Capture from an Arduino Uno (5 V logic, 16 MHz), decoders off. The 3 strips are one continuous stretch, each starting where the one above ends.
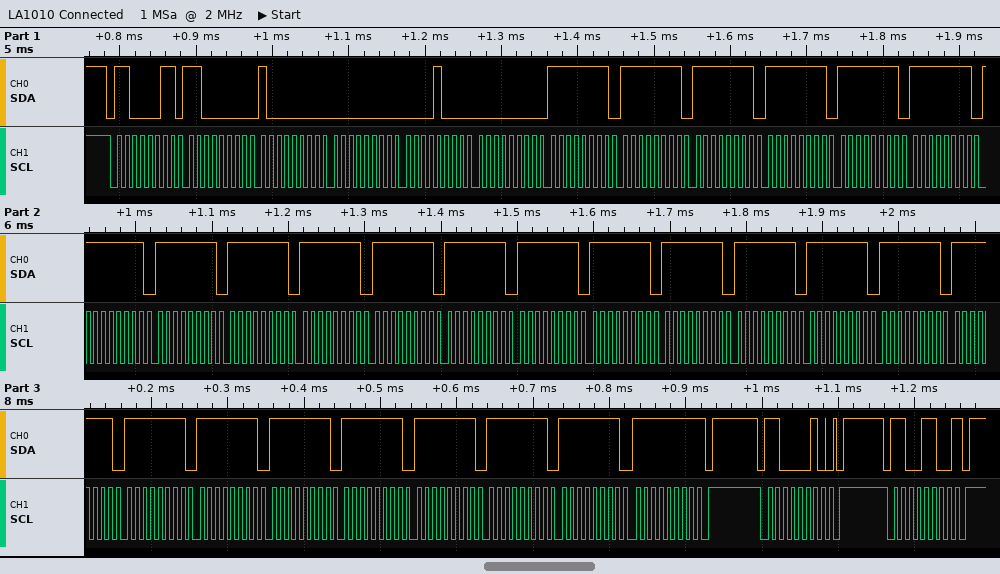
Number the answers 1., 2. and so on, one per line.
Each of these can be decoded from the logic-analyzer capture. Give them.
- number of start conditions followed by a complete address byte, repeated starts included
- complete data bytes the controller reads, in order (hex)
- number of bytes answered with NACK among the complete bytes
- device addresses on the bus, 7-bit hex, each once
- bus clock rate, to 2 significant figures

1. 3
2. C0 80 00 08 00 FF FF FF FF FF FF FF FF FF FF FF FF FF FF FF FF FF FF FF FF FF FF FF FF FF FF FF
3. 2
4. 0x61 0x66
5. 100 kHz
